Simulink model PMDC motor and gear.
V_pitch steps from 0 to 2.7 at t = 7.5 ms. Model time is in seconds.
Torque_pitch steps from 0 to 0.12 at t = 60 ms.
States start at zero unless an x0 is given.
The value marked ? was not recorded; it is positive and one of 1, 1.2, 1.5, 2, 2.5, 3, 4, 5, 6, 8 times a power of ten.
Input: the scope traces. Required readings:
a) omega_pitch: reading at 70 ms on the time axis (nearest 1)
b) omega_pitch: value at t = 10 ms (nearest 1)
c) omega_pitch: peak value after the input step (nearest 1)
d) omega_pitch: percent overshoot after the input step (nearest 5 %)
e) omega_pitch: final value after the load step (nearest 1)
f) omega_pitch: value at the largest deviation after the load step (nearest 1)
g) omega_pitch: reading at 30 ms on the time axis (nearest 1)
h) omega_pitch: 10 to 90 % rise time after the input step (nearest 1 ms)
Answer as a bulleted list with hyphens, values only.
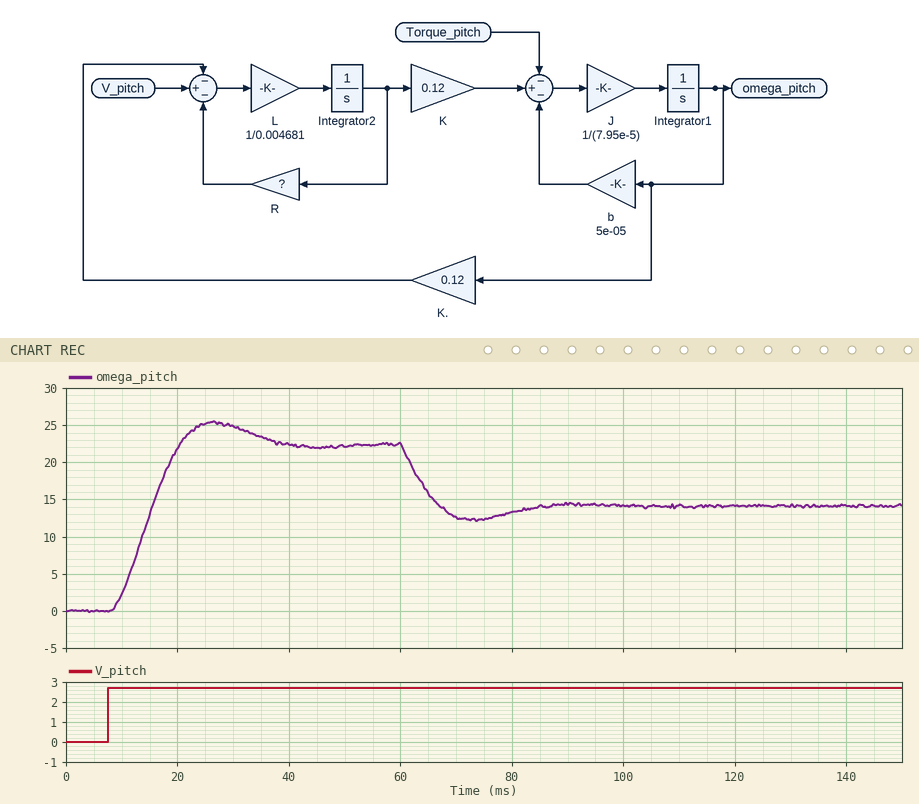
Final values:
- 13
- 2
- 25
- 15 %
- 14
- 12
- 25
- 9 ms
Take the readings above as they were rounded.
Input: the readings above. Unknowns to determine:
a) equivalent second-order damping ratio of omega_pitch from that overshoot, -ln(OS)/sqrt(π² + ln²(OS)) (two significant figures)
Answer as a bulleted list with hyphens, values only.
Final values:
- 0.52
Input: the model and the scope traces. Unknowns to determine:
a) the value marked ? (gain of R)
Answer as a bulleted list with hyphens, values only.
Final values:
- 1
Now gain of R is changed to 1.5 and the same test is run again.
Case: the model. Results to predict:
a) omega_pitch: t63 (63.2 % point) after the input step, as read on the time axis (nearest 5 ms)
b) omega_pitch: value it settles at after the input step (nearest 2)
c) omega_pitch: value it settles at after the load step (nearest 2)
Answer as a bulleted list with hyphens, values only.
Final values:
- 15 ms
- 22
- 10
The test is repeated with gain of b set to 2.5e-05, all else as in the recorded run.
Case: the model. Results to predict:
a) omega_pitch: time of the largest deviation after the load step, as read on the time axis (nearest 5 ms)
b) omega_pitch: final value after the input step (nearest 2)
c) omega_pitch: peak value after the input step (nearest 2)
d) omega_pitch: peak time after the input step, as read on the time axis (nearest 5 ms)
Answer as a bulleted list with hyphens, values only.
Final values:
- 75 ms
- 22
- 26
- 25 ms
